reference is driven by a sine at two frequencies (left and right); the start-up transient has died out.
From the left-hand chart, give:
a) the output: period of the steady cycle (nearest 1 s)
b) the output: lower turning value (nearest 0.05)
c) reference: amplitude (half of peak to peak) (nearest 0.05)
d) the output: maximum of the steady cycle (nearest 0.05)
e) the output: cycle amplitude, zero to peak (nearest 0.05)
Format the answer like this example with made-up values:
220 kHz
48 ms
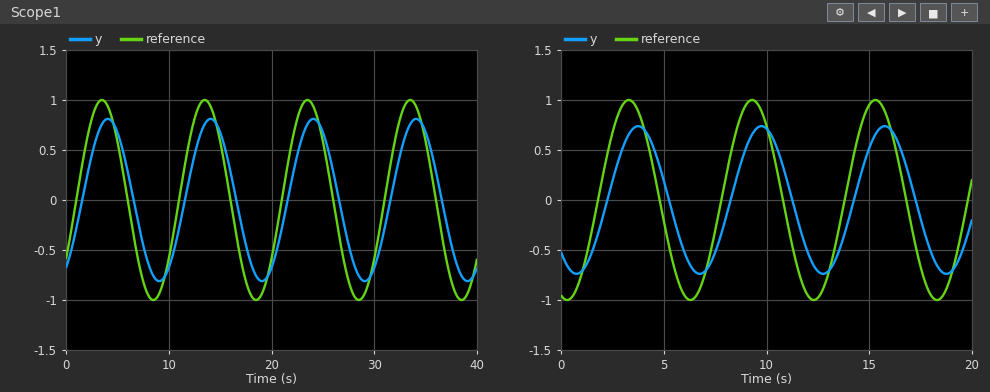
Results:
10 s
-0.80
1.00
0.80
0.80
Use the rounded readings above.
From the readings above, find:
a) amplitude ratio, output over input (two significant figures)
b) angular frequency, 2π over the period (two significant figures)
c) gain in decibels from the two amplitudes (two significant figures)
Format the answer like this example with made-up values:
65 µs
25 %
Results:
0.80
0.63 rad/s
-1.9 dB
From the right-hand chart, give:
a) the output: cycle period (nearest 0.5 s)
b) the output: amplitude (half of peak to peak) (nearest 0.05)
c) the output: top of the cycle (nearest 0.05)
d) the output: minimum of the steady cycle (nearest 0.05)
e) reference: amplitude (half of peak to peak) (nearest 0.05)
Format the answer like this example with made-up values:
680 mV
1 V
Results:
6.0 s
0.75
0.75
-0.75
1.00
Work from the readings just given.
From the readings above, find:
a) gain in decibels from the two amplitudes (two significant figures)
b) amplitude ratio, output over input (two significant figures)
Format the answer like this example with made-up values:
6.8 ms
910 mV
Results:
-2.5 dB
0.75
